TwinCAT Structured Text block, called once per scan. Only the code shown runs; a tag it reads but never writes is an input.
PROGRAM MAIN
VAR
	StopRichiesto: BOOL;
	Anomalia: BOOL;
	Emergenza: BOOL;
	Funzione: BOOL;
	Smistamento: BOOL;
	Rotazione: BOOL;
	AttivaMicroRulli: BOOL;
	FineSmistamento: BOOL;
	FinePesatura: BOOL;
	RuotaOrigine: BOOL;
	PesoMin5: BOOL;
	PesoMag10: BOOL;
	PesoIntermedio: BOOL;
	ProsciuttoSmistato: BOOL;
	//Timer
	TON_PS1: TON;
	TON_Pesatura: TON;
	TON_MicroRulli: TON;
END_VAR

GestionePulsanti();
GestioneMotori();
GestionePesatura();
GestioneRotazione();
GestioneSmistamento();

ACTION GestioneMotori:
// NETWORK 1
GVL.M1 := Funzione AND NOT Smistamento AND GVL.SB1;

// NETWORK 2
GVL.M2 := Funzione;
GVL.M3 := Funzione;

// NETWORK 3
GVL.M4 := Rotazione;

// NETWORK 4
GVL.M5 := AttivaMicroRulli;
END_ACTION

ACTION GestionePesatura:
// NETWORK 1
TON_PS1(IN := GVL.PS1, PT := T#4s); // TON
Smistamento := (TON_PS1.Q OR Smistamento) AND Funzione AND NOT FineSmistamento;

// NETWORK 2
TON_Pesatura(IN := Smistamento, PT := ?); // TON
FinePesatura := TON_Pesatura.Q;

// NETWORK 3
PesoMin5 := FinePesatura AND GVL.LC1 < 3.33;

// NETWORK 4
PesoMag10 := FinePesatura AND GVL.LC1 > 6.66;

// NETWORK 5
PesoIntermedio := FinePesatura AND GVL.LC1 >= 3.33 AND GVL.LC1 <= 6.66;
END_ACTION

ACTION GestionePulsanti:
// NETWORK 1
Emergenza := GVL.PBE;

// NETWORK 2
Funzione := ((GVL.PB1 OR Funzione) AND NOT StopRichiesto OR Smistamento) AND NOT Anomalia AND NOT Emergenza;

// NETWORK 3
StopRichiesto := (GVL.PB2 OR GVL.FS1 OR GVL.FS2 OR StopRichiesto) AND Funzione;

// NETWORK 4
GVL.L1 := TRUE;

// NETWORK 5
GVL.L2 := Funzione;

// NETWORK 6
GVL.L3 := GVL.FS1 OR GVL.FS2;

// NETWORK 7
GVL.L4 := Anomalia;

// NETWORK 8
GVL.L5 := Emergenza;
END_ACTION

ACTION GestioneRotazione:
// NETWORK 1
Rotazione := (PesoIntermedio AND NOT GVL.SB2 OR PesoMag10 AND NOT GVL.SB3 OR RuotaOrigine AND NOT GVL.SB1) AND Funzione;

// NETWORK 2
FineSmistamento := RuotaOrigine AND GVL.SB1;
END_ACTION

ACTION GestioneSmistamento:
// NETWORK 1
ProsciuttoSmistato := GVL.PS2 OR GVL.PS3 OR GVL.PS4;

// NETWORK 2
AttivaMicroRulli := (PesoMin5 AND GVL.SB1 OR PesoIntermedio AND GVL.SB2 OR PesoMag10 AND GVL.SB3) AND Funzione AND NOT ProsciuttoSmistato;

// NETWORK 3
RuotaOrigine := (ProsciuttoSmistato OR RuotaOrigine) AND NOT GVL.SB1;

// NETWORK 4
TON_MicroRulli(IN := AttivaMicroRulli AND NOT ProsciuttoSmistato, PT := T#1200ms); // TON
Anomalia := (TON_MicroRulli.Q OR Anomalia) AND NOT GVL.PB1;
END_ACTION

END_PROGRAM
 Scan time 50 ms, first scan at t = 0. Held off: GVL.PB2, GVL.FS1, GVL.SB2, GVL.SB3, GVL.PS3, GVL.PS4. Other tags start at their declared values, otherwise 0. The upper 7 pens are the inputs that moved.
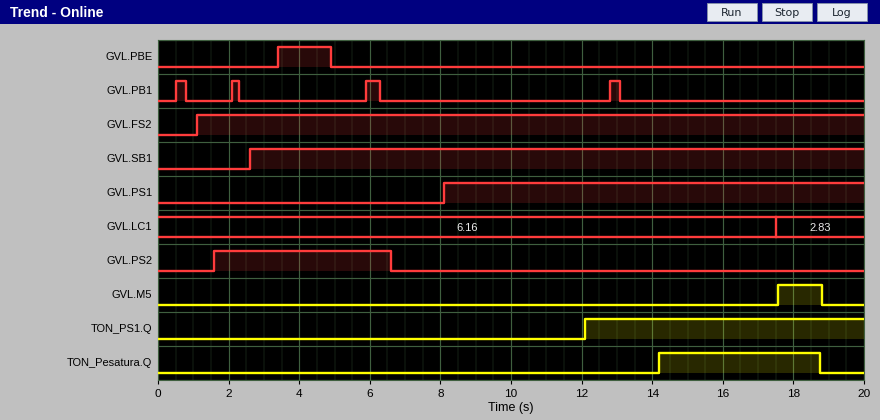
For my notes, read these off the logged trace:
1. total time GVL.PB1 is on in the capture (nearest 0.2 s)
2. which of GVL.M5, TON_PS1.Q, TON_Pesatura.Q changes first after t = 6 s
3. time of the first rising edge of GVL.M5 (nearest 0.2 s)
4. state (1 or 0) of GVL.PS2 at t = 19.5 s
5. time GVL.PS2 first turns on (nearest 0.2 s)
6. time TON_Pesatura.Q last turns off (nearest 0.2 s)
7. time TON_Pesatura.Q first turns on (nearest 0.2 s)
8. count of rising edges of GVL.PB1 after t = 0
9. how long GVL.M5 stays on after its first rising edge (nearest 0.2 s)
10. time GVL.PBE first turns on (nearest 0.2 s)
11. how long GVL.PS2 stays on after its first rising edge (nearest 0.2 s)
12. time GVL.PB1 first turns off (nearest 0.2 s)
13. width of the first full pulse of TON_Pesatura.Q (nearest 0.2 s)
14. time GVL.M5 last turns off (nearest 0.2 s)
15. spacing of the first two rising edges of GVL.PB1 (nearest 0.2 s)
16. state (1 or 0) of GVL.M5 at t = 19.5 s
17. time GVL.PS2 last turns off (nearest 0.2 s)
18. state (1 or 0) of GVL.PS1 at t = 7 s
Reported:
1.2 s
TON_PS1.Q
17.6 s
0
1.6 s
18.8 s
14.2 s
4
1.2 s
3.4 s
5.0 s
0.8 s
4.6 s
18.8 s
1.6 s
0
6.6 s
0
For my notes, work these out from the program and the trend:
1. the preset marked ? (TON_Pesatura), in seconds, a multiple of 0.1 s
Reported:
1.4 s
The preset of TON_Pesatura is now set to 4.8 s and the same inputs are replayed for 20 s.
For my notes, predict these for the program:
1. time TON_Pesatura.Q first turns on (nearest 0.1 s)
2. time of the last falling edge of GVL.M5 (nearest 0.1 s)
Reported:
17.6 s
18.9 s
